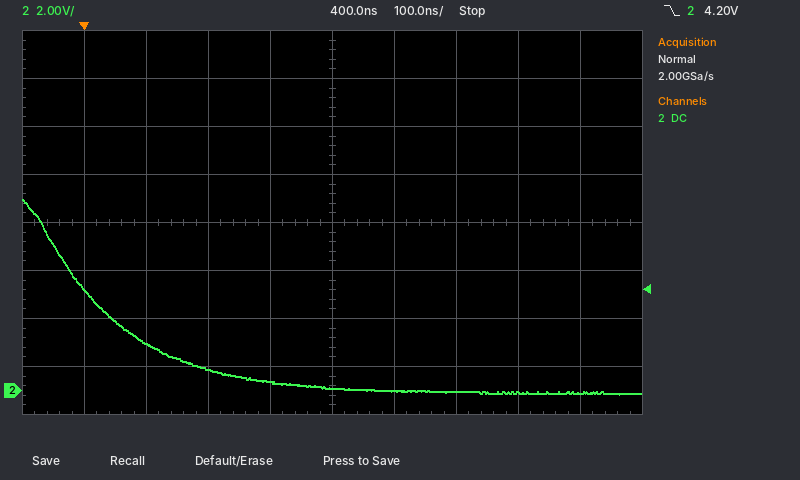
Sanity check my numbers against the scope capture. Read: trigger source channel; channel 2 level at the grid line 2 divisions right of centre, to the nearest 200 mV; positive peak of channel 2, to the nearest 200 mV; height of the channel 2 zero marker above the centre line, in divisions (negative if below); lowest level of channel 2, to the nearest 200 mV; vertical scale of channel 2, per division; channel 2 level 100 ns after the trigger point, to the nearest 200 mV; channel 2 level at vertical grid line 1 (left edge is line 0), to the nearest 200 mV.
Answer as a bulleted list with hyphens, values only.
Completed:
- channel 2
- 0.0 V
- 8.0 V
- -3.5 div
- -200 mV
- 2 V
- 2.0 V
- 4.2 V
